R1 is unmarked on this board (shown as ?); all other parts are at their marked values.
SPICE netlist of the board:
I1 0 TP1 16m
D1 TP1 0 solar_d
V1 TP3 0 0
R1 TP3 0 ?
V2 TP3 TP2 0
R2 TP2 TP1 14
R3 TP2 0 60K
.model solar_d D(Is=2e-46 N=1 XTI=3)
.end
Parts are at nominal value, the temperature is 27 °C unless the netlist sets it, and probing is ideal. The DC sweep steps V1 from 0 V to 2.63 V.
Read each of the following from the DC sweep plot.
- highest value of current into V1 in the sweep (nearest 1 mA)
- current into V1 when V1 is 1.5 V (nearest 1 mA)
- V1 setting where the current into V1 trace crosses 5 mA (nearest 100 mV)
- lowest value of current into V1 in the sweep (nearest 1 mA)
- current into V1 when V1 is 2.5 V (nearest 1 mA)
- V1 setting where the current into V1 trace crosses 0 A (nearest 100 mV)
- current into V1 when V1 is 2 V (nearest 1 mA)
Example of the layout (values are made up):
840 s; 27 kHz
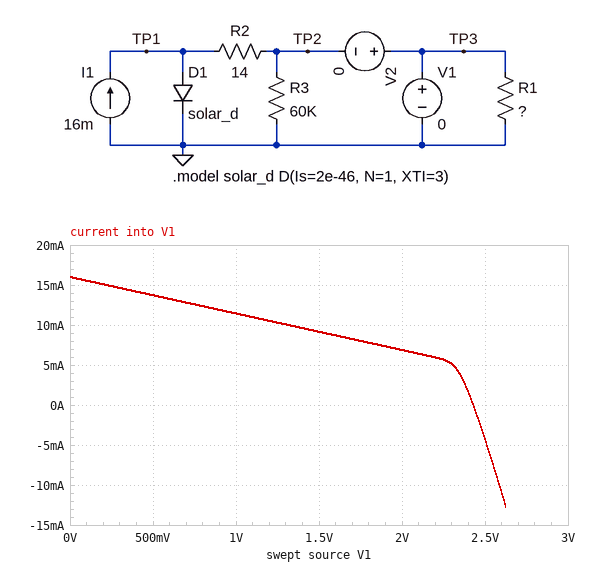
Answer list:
16 mA; 9 mA; 2.3 V; -13 mA; -4 mA; 2.4 V; 7 mA
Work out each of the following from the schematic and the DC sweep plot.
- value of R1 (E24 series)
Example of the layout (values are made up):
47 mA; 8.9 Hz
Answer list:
220 Ω
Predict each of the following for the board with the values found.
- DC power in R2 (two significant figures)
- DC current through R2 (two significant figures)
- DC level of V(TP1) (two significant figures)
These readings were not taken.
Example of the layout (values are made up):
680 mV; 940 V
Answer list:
3.6 mW; 16 mA; 220 mV
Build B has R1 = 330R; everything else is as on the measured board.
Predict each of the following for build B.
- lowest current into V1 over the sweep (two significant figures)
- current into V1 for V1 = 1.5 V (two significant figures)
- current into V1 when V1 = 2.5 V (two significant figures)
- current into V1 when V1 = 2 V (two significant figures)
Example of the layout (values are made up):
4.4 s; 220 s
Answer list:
-9.0 mA; 11 mA; -510 µA; 9.9 mA
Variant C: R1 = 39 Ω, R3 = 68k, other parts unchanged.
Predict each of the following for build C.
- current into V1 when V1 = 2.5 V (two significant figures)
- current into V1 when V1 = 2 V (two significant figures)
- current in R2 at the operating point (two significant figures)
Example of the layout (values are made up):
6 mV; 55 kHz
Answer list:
-57 mA; -35 mA; 16 mA
